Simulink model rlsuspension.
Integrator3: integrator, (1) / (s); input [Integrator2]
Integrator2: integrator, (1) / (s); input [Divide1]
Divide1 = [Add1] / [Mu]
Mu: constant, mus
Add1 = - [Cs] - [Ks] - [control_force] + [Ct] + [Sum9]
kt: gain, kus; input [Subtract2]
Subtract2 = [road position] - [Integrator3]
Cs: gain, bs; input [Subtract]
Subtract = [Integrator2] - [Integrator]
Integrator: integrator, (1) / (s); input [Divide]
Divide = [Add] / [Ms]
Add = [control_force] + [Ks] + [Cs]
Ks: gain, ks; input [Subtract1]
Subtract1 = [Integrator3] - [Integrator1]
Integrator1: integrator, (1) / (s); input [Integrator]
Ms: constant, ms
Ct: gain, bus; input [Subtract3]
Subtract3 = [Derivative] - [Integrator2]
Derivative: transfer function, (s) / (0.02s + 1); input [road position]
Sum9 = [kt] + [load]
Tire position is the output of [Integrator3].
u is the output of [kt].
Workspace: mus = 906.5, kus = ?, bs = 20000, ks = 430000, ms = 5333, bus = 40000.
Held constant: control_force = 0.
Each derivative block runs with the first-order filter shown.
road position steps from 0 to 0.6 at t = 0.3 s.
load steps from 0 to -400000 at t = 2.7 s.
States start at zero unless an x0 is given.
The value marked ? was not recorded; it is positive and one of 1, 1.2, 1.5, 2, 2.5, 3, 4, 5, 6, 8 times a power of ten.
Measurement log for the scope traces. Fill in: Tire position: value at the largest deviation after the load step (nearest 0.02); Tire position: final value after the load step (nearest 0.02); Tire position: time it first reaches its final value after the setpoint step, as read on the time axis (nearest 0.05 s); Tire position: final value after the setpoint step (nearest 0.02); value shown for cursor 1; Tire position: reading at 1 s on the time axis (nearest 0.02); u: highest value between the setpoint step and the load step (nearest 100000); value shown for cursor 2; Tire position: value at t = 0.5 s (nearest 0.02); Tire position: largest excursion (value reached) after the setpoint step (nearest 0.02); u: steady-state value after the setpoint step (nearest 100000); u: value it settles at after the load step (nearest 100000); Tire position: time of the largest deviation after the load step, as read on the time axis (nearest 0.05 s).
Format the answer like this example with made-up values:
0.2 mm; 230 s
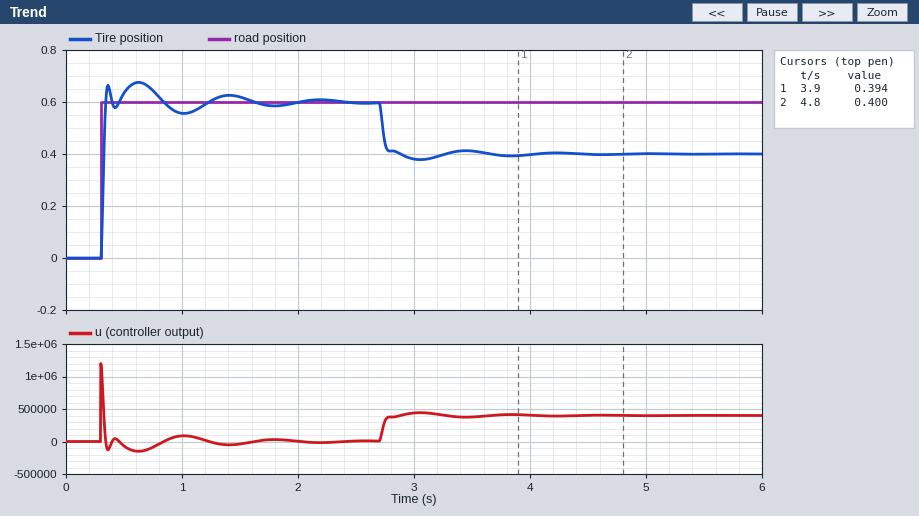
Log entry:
0.38; 0.40; 0.35 s; 0.60; 0.394; 0.56; 1200000; 0.400; 0.64; 0.68; 0; 400000; 3.05 s
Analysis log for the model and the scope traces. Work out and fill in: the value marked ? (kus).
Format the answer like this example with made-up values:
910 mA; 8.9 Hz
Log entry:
2e+06
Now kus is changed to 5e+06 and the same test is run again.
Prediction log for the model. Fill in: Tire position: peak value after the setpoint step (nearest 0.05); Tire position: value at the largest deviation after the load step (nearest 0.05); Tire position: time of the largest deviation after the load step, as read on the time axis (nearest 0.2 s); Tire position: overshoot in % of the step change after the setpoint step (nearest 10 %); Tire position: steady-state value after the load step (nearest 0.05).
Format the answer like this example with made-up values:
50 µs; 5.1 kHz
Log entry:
0.80; 0.50; 2.8 s; 30 %; 0.50
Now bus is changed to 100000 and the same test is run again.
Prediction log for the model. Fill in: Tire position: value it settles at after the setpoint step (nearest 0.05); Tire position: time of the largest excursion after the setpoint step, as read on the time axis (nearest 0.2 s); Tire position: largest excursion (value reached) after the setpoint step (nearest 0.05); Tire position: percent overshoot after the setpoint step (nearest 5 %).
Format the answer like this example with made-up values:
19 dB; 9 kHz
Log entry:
0.60; 0.6 s; 0.65; 10 %
